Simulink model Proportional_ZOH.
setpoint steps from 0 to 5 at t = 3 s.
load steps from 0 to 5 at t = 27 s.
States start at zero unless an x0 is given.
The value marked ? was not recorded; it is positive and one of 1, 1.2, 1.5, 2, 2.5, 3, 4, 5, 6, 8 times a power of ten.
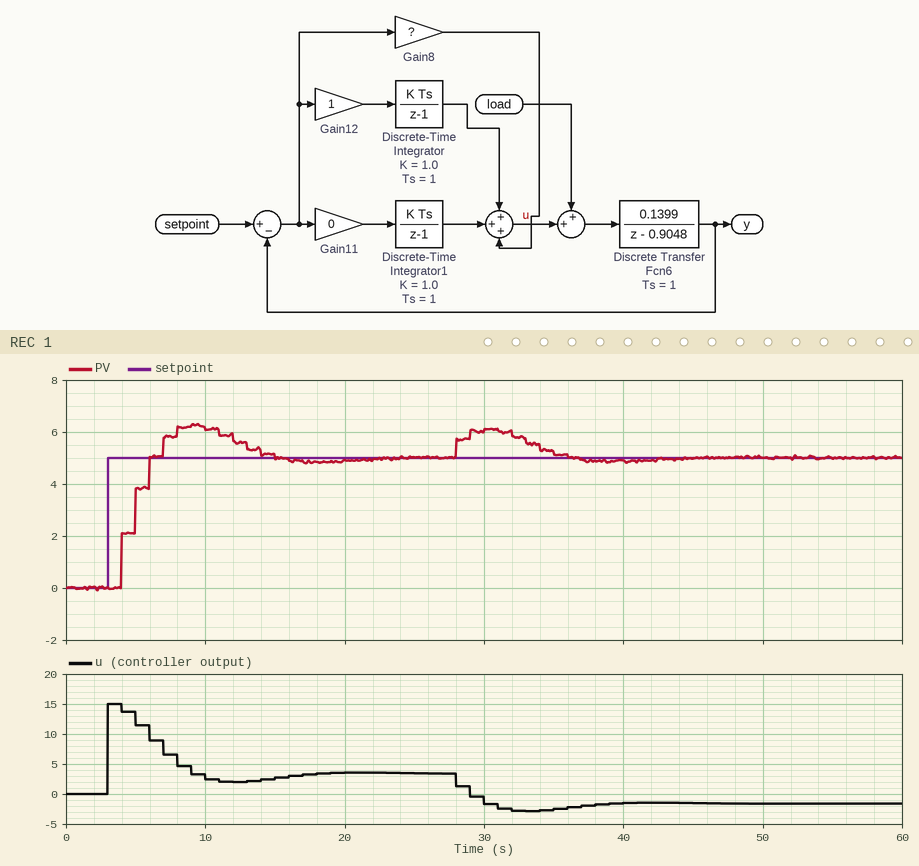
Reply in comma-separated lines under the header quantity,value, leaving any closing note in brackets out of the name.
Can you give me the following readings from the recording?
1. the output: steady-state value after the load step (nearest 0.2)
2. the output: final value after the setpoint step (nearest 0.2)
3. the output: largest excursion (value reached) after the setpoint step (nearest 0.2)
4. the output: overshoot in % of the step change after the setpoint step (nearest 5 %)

quantity,value
the output: steady-state value after the load step,5.0
the output: final value after the setpoint step,5.0
the output: largest excursion (value reached) after the setpoint step,6.2
the output: overshoot in % of the step change after the setpoint step,25 %
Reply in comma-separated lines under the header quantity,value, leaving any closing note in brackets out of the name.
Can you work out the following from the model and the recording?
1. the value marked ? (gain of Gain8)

quantity,value
the value marked ?,3
